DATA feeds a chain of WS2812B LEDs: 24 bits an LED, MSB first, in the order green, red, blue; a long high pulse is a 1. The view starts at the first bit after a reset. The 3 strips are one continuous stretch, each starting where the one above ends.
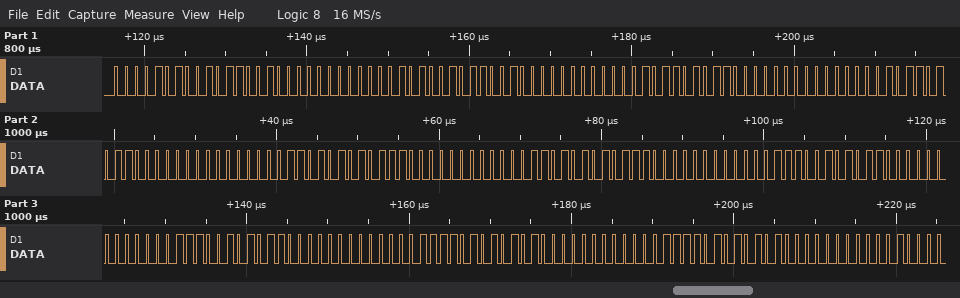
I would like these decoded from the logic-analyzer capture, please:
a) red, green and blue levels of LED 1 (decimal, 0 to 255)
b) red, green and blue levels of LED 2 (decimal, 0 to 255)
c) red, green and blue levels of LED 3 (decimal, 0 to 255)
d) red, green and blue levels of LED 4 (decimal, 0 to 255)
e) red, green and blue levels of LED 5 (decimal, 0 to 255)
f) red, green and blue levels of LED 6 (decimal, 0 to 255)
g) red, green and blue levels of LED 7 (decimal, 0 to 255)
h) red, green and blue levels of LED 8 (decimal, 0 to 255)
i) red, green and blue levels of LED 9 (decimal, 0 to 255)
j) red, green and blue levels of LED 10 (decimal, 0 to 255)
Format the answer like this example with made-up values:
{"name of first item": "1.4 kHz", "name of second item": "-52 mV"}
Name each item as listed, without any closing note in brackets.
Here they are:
{"red, green and blue levels of LED 1": "89, 10, 0", "red, green and blue levels of LED 2": "89, 10, 0", "red, green and blue levels of LED 3": "88, 11, 0", "red, green and blue levels of LED 4": "88, 11, 0", "red, green and blue levels of LED 5": "87, 13, 0", "red, green and blue levels of LED 6": "87, 13, 0", "red, green and blue levels of LED 7": "86, 14, 0", "red, green and blue levels of LED 8": "86, 14, 0", "red, green and blue levels of LED 9": "85, 15, 0", "red, green and blue levels of LED 10": "85, 15, 0"}
